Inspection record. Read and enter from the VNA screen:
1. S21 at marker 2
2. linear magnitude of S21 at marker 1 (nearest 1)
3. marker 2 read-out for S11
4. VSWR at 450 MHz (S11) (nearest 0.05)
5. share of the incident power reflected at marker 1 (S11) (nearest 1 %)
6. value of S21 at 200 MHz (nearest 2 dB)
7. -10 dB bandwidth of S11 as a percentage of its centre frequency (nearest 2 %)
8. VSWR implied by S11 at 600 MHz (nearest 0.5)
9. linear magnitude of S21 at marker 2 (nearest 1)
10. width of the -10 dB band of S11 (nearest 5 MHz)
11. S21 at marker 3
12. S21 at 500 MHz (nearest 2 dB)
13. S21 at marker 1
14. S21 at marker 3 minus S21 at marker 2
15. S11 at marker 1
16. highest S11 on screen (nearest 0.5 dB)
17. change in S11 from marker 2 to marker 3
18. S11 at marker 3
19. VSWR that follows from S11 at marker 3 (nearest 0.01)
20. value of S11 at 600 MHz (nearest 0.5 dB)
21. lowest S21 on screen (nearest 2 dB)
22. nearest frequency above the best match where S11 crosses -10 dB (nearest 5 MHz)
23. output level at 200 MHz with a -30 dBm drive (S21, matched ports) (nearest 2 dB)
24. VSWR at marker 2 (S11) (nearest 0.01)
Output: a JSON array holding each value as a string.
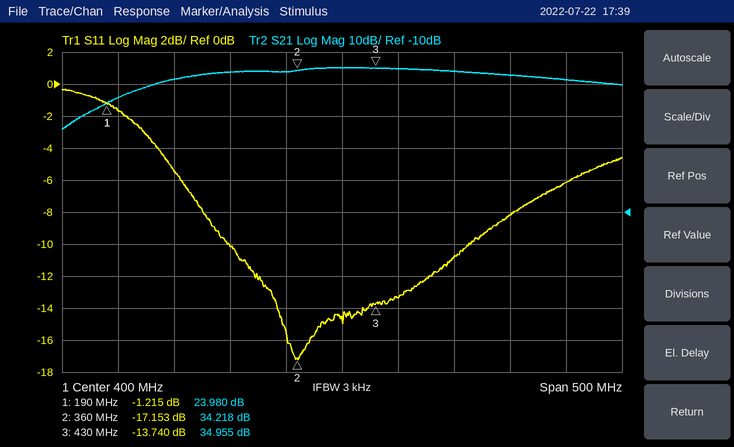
["34.218 dB", "16", "-17.153 dB", "1.55", "76 %", "26 dB", "52 %", "3.0", "51", "215 MHz", "34.955 dB", "34 dB", "23.980 dB", "0.737 dB", "-1.215 dB", "-0.5 dB", "3.413 dB", "-13.740 dB", "1.52", "-6.0 dB", "16 dB", "515 MHz", "-4 dBm", "1.32"]
